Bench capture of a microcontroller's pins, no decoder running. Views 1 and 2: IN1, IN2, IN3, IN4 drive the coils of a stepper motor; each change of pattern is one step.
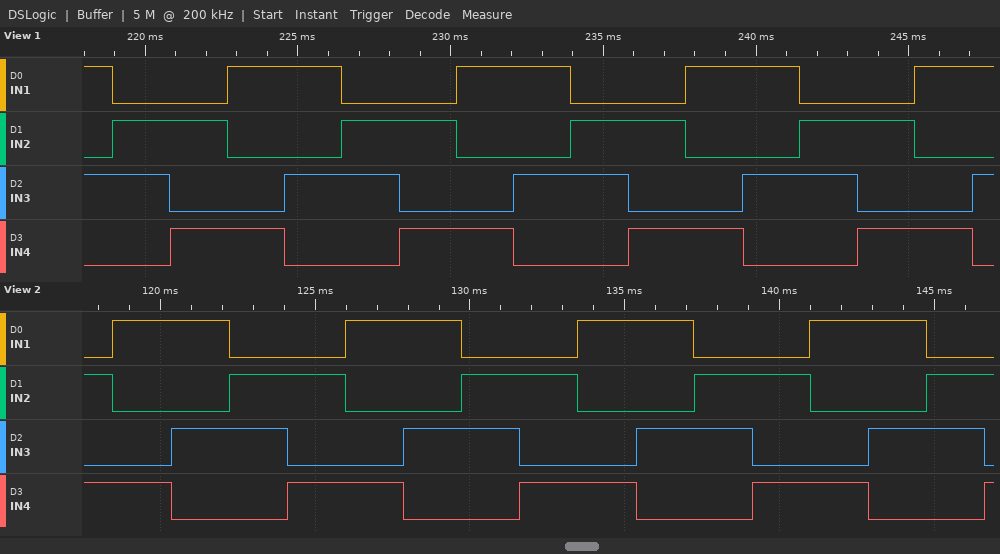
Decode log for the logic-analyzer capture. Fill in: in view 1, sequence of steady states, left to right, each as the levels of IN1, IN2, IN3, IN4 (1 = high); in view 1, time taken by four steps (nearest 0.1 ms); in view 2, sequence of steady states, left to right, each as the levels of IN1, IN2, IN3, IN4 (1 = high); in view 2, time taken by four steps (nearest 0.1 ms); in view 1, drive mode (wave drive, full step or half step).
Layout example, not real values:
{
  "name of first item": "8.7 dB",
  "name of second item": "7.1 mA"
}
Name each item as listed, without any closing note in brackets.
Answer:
{
  "in view 1, sequence of steady states, left to right, each as the levels of IN1, IN2, IN3, IN4": "1010 0110 0101 1001 1010 0110 0101 1001 1010 0110 0101 1001 1010 0110 0101 1001 1010",
  "in view 1, time taken by four steps": "7.5 ms",
  "in view 2, sequence of steady states, left to right, each as the levels of IN1, IN2, IN3, IN4": "0101 1001 1010 0110 0101 1001 1010 0110 0101 1001 1010 0110 0101 1001 1010 0110 0101",
  "in view 2, time taken by four steps": "7.5 ms",
  "in view 1, drive mode": "full step"
}
